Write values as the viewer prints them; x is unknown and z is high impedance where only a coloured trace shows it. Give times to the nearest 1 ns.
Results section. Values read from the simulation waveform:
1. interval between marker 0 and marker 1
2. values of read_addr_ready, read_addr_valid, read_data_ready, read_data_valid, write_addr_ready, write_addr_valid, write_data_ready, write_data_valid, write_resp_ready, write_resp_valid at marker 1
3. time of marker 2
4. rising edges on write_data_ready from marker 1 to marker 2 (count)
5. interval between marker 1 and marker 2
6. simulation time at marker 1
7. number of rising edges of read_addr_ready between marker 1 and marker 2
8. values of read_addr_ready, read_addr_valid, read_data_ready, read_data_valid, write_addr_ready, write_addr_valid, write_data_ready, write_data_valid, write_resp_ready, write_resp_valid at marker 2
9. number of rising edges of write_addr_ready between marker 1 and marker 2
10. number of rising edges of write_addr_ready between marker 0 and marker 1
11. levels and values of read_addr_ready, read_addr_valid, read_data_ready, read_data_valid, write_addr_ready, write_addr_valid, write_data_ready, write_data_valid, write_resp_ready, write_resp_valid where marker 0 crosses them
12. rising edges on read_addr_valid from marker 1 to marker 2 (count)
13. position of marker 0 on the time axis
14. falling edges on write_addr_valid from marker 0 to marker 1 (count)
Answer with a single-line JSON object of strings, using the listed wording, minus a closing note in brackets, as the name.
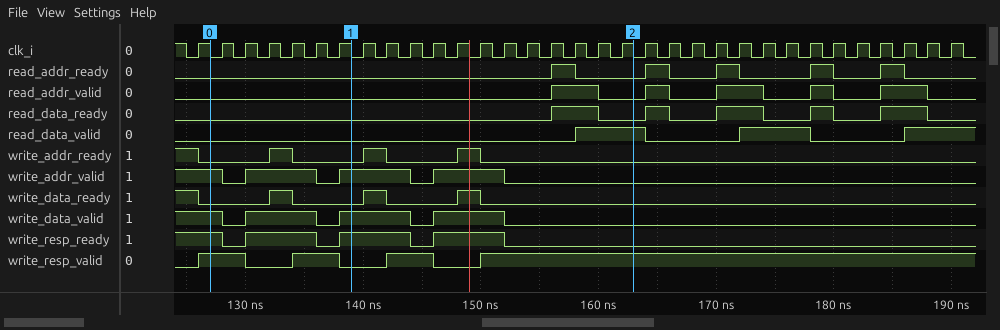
{"interval between marker 0 and marker 1": "12 ns", "values of read_addr_ready, read_addr_valid, read_data_ready, read_data_valid, write_addr_ready, write_addr_valid, write_data_ready, write_data_valid, write_resp_ready, write_resp_valid at marker 1": "read_addr_ready=0, read_addr_valid=0, read_data_ready=0, read_data_valid=0, write_addr_ready=0, write_addr_valid=1, write_data_ready=0, write_data_valid=1, write_resp_ready=1, write_resp_valid=0", "time of marker 2": "163 ns", "rising edges on write_data_ready from marker 1 to marker 2": "2", "interval between marker 1 and marker 2": "24 ns", "simulation time at marker 1": "139 ns", "number of rising edges of read_addr_ready between marker 1 and marker 2": "1", "values of read_addr_ready, read_addr_valid, read_data_ready, read_data_valid, write_addr_ready, write_addr_valid, write_data_ready, write_data_valid, write_resp_ready, write_resp_valid at marker 2": "read_addr_ready=0, read_addr_valid=0, read_data_ready=0, read_data_valid=1, write_addr_ready=0, write_addr_valid=0, write_data_ready=0, write_data_valid=0, write_resp_ready=0, write_resp_valid=1", "number of rising edges of write_addr_ready between marker 1 and marker 2": "2", "number of rising edges of write_addr_ready between marker 0 and marker 1": "1", "levels and values of read_addr_ready, read_addr_valid, read_data_ready, read_data_valid, write_addr_ready, write_addr_valid, write_data_ready, write_data_valid, write_resp_ready, write_resp_valid where marker 0 crosses them": "read_addr_ready=0, read_addr_valid=0, read_data_ready=0, read_data_valid=0, write_addr_ready=0, write_addr_valid=1, write_data_ready=0, write_data_valid=1, write_resp_ready=1, write_resp_valid=1", "rising edges on read_addr_valid from marker 1 to marker 2": "1", "position of marker 0 on the time axis": "127 ns", "falling edges on write_addr_valid from marker 0 to marker 1": "2"}
